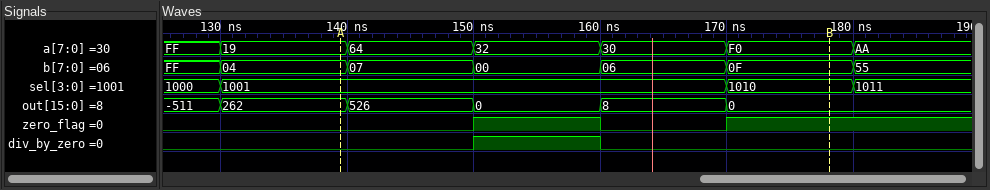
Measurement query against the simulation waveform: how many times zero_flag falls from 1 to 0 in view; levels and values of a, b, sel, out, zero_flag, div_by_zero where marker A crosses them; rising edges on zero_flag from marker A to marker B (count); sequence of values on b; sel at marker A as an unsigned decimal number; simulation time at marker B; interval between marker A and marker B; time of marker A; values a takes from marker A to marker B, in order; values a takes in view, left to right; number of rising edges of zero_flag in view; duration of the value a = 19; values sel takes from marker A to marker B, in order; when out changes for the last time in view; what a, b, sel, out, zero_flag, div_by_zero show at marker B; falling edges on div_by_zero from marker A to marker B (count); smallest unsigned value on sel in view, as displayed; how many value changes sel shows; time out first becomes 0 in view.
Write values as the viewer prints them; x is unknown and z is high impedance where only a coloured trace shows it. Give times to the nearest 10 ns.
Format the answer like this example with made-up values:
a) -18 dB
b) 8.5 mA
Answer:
a) 1
b) a=19, b=04, sel=1001, out=262, zero_flag=0, div_by_zero=0
c) 2
d) FF, 04, 07, 00, 06, 0F, 55
e) 9
f) 180 ns
g) 40 ns
h) 140 ns
i) 19, 64, 32, 30, F0
j) FF, 19, 64, 32, 30, F0, AA
k) 2
l) 10 ns
m) 1001, 1010
n) 170 ns
o) a=F0, b=0F, sel=1010, out=0, zero_flag=1, div_by_zero=0
p) 1
q) 1000
r) 3
s) 150 ns
